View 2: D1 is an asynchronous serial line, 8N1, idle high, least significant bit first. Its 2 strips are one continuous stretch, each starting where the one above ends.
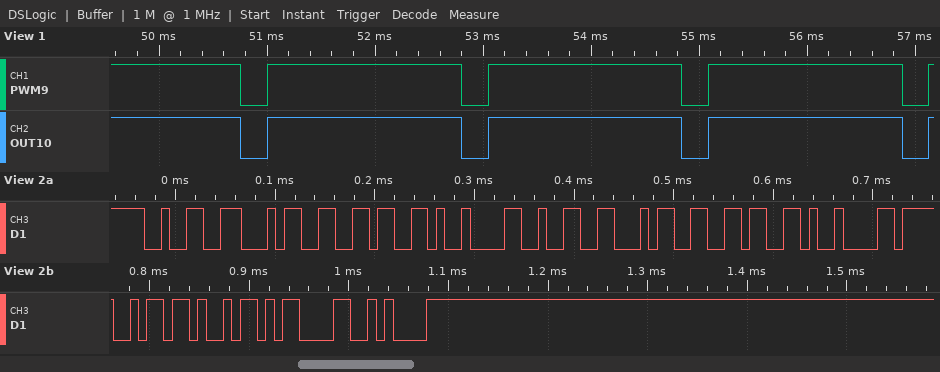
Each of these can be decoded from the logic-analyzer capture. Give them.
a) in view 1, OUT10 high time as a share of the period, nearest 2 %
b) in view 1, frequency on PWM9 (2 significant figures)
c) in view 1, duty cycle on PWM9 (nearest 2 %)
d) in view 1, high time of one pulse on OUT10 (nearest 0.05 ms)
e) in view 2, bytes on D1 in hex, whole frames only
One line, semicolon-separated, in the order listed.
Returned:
88 %; 490 Hz; 88 %; 1.80 ms; 32 34 36 09 32 34 36 09 4F 4B 0D 0A
